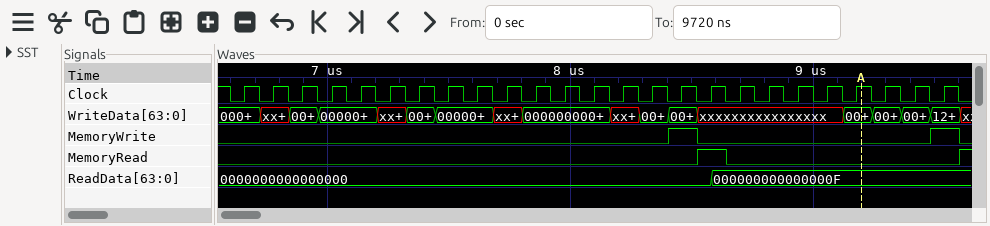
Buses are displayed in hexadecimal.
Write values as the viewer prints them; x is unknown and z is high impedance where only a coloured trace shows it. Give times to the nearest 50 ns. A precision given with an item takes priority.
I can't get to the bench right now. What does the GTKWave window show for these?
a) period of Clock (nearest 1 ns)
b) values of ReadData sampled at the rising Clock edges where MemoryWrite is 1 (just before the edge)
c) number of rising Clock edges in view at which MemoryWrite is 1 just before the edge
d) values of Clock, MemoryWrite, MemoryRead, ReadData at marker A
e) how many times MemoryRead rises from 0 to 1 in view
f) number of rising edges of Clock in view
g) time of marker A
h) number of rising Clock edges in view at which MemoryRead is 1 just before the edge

120 ns
0000000000000000, 000000000000000F
2
Clock=1, MemoryWrite=0, MemoryRead=0, ReadData=000000000000000F
2
25
9200 ns
1
